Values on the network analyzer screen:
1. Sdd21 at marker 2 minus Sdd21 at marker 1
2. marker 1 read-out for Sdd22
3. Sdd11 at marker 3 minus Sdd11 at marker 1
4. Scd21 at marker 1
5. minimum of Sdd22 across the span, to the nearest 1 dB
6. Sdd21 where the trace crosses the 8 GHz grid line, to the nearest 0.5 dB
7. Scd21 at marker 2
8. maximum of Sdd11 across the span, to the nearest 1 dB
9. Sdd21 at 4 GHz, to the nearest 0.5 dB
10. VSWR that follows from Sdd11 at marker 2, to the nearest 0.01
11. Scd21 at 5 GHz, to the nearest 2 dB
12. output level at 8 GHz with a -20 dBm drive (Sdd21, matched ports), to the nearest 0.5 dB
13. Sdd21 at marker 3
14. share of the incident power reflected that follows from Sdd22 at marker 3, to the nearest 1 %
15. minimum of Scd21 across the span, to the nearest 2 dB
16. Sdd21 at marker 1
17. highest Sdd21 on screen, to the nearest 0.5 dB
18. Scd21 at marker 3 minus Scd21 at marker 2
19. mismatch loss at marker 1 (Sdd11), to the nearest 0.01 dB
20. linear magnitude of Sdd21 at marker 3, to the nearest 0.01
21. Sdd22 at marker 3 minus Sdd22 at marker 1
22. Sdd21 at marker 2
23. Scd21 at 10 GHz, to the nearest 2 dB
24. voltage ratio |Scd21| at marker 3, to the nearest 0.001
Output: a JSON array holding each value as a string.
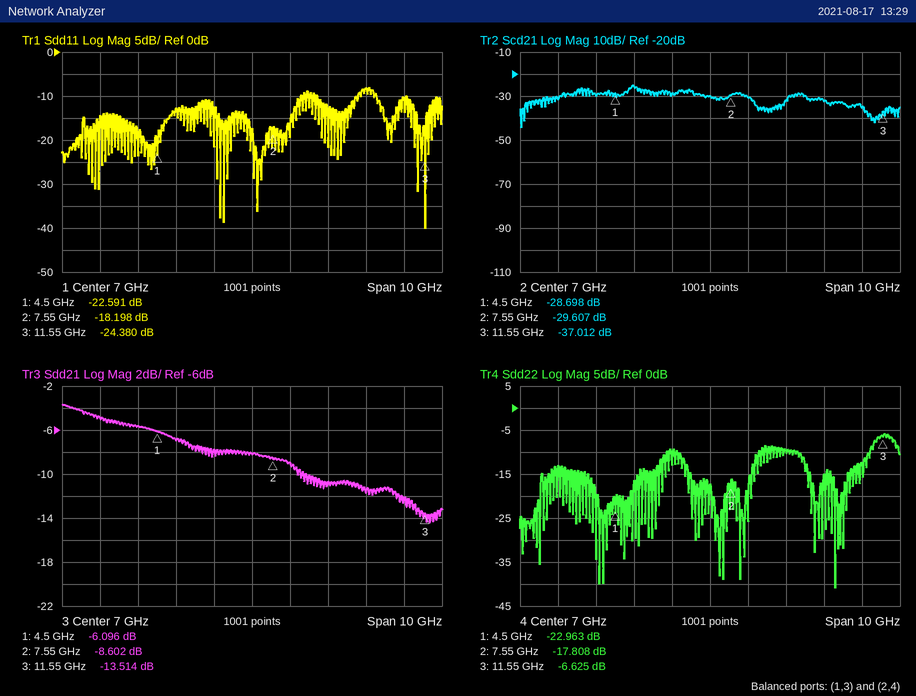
["-2.506 dB", "-22.963 dB", "-1.789 dB", "-28.698 dB", "-41 dB", "-9.0 dB", "-29.607 dB", "-8 dB", "-5.5 dB", "1.28", "-26 dB", "-29.0 dBm", "-13.514 dB", "22 %", "-44 dB", "-6.096 dB", "-3.5 dB", "-7.405 dB", "0.02 dB", "0.21", "16.338 dB", "-8.602 dB", "-32 dB", "0.014"]
